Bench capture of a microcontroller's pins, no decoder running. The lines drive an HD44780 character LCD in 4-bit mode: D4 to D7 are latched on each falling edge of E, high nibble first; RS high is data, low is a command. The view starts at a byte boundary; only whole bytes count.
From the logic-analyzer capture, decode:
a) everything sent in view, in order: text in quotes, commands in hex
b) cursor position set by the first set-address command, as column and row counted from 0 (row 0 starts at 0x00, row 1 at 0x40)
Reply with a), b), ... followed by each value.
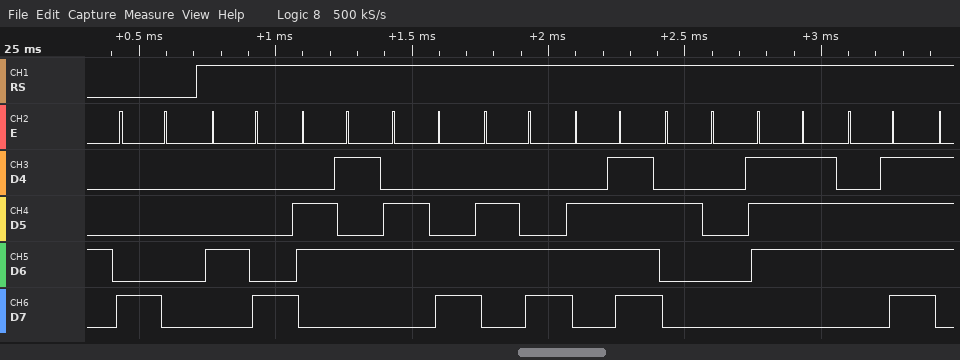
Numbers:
a) 0x80 "Hello wo"
b) column 0, row 0
